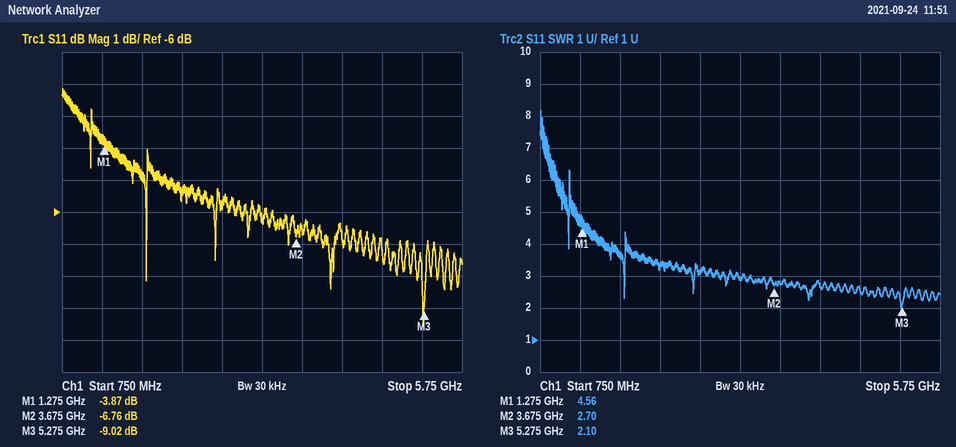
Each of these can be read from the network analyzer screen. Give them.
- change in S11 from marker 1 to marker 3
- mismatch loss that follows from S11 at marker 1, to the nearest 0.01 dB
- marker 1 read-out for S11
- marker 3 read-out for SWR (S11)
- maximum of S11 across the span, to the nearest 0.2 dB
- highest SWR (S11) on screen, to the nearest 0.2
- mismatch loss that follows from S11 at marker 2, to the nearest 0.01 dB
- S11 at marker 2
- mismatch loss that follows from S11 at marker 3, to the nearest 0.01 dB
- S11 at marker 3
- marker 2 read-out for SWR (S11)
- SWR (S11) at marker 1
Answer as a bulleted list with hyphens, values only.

- -5.15 dB
- 2.29 dB
- -3.87 dB
- 2.10
- -2.2 dB
- 8.2
- 1.03 dB
- -6.76 dB
- 0.58 dB
- -9.02 dB
- 2.70
- 4.56
